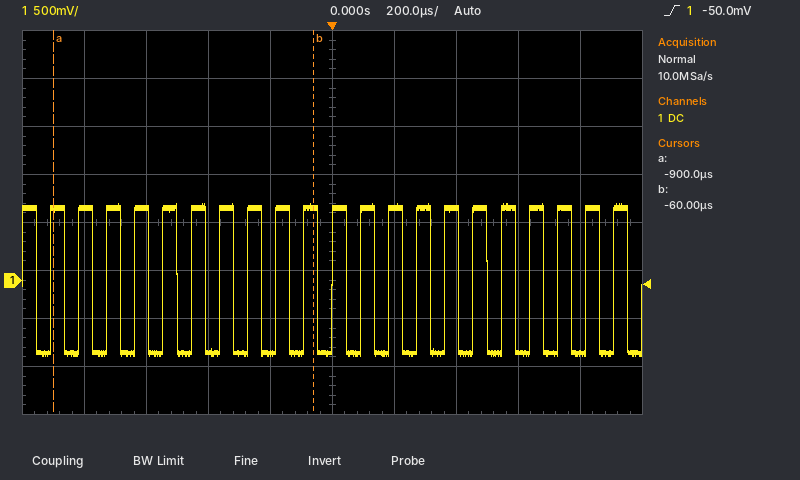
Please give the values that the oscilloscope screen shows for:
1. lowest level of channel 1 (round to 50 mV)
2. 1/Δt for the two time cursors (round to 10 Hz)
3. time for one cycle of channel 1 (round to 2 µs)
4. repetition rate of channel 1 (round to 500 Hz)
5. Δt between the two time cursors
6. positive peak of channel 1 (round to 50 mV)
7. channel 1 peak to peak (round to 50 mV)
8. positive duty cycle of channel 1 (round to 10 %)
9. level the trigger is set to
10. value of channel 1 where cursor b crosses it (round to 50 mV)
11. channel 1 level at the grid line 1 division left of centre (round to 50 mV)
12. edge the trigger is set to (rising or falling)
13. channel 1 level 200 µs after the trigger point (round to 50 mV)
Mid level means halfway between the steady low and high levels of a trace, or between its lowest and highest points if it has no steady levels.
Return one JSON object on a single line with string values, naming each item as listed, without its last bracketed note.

{"lowest level of channel 1": "-800 mV", "1/Δt for the two time cursors": "1.19 kHz", "time for one cycle of channel 1": "90 µs", "repetition rate of channel 1": "11.0 kHz", "Δt between the two time cursors": "840 µs", "positive peak of channel 1": "800 mV", "channel 1 peak to peak": "1.60 V", "positive duty cycle of channel 1": "50 %", "level the trigger is set to": "-50.0 mV", "value of channel 1 where cursor b crosses it": "750 mV", "channel 1 level at the grid line 1 division left of centre": "-750 mV", "edge the trigger is set to": "rising", "channel 1 level 200 µs after the trigger point": "750 mV"}
